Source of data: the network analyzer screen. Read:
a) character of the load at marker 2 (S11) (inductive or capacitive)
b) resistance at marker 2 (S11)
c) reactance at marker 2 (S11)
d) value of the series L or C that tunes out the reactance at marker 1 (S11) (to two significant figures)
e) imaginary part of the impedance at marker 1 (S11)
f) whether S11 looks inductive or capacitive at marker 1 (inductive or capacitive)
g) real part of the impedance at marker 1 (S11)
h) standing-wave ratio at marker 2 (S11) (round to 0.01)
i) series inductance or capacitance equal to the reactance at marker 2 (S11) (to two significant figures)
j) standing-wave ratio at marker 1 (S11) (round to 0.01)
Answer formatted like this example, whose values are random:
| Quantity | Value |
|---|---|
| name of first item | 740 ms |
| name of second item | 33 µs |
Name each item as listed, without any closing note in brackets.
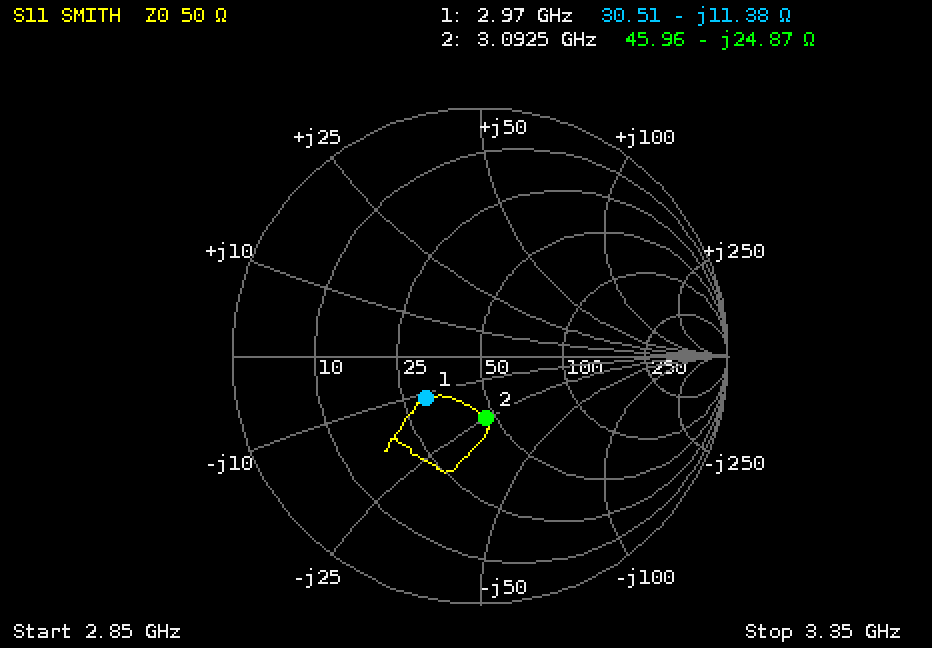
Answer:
| Quantity | Value |
|---|---|
| character of the load at marker 2 (S11) | capacitive |
| resistance at marker 2 | 45.96 Ω |
| reactance at marker 2 | -24.87 Ω |
| value of the series L or C that tunes out the reactance at marker 1 (S11) | 610 pH |
| imaginary part of the impedance at marker 1 | -11.38 Ω |
| whether S11 looks inductive or capacitive at marker 1 | capacitive |
| real part of the impedance at marker 1 | 30.51 Ω |
| standing-wave ratio at marker 2 (S11) | 1.68 |
| series inductance or capacitance equal to the reactance at marker 2 (S11) | 2.1 pF |
| standing-wave ratio at marker 1 (S11) | 1.77 |
